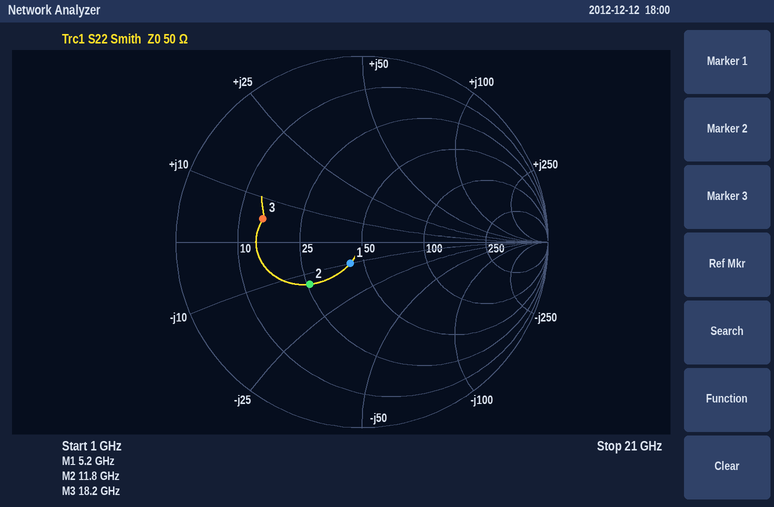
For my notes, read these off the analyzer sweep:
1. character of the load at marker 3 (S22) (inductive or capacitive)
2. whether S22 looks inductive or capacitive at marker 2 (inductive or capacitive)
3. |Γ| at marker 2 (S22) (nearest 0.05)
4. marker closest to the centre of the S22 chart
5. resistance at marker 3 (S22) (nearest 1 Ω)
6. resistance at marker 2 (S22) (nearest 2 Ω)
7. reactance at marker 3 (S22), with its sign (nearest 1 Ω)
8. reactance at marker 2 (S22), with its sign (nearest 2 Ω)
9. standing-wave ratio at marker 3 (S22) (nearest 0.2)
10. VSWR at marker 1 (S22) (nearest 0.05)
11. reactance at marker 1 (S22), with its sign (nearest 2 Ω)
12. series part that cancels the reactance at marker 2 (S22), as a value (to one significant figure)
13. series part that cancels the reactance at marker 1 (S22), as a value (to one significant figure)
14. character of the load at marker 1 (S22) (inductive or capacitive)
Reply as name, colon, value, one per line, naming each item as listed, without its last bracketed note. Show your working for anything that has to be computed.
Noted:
character of the load at marker 3 (S22): inductive
whether S22 looks inductive or capacitive at marker 2: capacitive
|Γ| at marker 2 (S22): 0.35
marker closest to the centre of the S22 chart: marker 1
resistance at marker 3 (S22): 15 Ω
resistance at marker 2 (S22): 26 Ω
reactance at marker 3 (S22), with its sign: +5 Ω
reactance at marker 2 (S22), with its sign: -14 Ω
standing-wave ratio at marker 3 (S22): 3.4
VSWR at marker 1 (S22): 1.30
reactance at marker 1 (S22), with its sign: -10 Ω
series part that cancels the reactance at marker 2 (S22), as a value: L = 14 Ω/(2π × 11.8 GHz) ≈ 189 pH, so 200 pH to one significant figure
series part that cancels the reactance at marker 1 (S22), as a value: L = 10 Ω/(2π × 5.2 GHz) ≈ 306 pH, so 300 pH to one significant figure
character of the load at marker 1 (S22): capacitive
